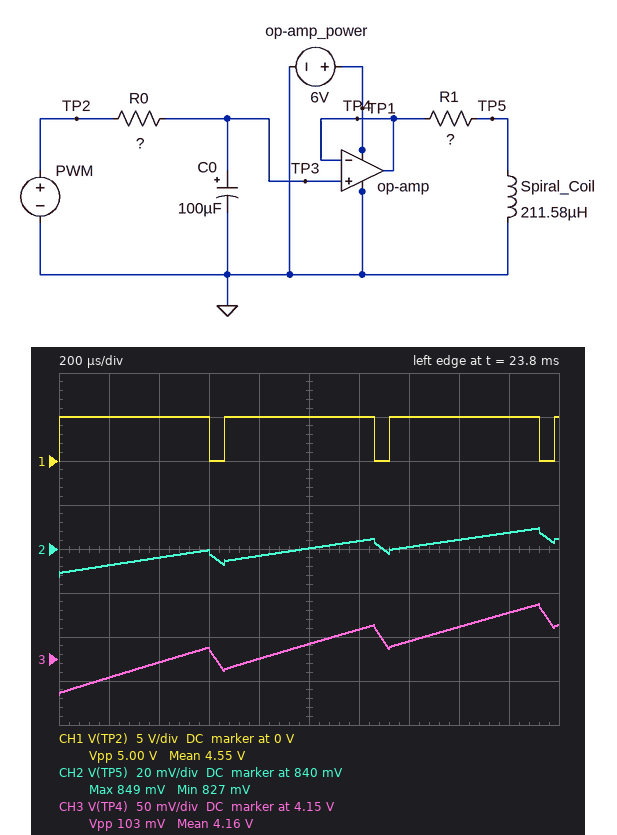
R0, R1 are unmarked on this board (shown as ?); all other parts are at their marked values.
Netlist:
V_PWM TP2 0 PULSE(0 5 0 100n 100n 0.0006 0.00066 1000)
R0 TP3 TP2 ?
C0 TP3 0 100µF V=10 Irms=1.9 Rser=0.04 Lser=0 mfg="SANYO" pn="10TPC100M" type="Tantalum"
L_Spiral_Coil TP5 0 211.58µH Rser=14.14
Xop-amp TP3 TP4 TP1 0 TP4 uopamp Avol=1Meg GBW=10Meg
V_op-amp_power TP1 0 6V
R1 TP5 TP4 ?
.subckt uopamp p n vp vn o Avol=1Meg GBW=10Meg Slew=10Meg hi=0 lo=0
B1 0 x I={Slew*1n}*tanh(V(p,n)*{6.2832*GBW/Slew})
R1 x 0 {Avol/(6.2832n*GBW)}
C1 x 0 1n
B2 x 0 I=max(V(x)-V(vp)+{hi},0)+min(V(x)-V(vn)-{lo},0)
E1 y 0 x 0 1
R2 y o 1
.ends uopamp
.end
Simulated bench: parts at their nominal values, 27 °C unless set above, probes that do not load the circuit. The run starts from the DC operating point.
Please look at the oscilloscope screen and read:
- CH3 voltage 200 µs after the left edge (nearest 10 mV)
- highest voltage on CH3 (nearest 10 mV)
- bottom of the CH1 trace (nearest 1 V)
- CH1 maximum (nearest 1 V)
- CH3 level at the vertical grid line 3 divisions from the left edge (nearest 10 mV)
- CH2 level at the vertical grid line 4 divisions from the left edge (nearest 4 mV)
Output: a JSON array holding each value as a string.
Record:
["4.13 V", "4.21 V", "0 V", "5 V", "4.16 V", "836 mV"]
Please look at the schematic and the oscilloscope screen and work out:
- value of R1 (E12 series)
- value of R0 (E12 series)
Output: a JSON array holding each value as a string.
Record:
["56 Ω", "100 Ω"]
